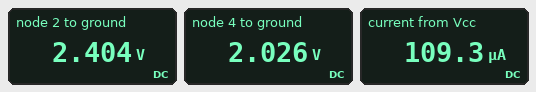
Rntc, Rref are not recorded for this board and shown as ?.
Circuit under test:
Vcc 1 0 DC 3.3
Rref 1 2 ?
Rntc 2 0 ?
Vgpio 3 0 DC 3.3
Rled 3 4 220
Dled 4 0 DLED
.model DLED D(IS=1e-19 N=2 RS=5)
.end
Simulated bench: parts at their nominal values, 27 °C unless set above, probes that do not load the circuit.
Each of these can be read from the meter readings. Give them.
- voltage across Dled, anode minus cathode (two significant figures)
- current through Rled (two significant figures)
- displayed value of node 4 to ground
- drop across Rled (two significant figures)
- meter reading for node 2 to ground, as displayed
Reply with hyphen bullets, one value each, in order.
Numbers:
- 2.0 V
- 5.8 mA
- 2.026 V
- 1.3 V
- 2.404 V
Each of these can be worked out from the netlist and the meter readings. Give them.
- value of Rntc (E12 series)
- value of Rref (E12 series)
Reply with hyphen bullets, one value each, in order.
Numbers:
- 22 kΩ
- 8.2 kΩ
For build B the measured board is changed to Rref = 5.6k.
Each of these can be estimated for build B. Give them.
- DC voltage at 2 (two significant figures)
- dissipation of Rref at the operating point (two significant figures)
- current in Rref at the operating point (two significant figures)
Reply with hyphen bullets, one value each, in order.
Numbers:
- 2.6 V
- 80 µW
- 120 µA
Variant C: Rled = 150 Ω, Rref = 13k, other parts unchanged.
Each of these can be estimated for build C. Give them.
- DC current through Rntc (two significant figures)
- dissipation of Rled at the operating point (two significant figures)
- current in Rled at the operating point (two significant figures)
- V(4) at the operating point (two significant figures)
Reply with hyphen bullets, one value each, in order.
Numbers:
- 94 µA
- 10 mW
- 8.3 mA
- 2.1 V
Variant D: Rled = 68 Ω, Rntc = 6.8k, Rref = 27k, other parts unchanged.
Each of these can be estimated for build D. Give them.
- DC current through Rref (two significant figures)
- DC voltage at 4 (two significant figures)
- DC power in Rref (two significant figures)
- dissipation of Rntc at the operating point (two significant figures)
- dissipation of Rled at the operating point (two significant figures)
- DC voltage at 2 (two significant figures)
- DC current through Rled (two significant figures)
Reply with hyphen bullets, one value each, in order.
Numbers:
- 98 µA
- 2.1 V
- 260 µW
- 65 µW
- 20 mW
- 660 mV
- 17 mA
